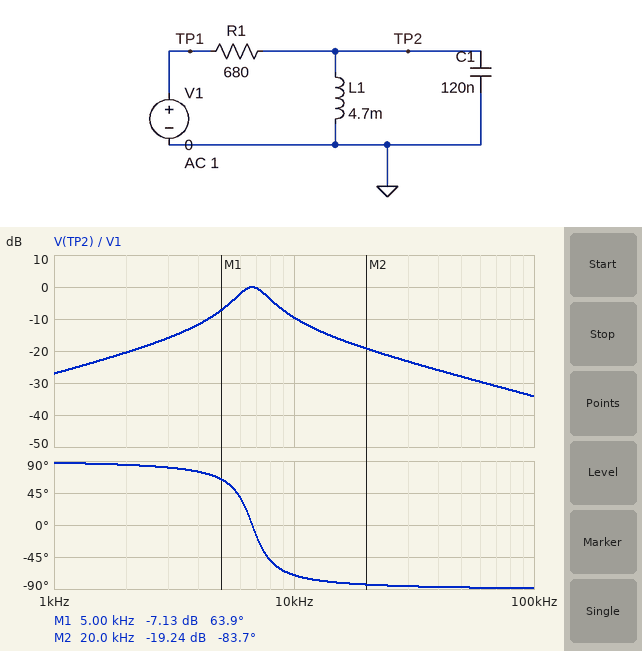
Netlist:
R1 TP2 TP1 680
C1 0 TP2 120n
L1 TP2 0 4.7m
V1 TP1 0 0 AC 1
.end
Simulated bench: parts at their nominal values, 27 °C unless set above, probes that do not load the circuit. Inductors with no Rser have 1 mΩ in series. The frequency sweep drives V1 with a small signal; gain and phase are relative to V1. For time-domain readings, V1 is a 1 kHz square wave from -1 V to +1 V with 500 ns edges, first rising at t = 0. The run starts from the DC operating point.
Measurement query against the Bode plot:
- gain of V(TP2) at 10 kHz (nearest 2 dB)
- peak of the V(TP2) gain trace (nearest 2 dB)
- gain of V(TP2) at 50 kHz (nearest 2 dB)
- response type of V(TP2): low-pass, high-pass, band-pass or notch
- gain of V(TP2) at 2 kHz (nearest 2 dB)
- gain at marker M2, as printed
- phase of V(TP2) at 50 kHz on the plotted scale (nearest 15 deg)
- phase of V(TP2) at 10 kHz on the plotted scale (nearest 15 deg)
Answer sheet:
-10 dB
0 dB
-28 dB
band-pass
-20 dB
-19.24 dB
-90 deg
-75 deg
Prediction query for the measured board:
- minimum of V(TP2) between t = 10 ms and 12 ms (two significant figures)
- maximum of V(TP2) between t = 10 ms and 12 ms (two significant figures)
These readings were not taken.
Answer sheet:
-480 mV
480 mV
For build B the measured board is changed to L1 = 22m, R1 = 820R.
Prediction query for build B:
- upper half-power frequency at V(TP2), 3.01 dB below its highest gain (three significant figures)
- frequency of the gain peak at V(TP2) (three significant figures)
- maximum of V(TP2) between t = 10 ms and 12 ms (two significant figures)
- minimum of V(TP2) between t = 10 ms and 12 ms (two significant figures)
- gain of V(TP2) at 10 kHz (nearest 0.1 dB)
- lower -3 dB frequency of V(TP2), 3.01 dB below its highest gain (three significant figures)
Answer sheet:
4.01 kHz
3.10 kHz
800 mV
-800 mV
-15.1 dB
2.39 kHz
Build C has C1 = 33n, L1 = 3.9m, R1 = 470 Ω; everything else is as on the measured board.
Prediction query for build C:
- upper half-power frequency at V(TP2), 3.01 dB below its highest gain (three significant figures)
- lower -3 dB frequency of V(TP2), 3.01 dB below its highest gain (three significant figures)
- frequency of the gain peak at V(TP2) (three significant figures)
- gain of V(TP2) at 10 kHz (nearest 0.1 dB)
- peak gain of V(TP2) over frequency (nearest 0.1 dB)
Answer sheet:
20.1 kHz
9.81 kHz
14.0 kHz
-2.8 dB
0 dB
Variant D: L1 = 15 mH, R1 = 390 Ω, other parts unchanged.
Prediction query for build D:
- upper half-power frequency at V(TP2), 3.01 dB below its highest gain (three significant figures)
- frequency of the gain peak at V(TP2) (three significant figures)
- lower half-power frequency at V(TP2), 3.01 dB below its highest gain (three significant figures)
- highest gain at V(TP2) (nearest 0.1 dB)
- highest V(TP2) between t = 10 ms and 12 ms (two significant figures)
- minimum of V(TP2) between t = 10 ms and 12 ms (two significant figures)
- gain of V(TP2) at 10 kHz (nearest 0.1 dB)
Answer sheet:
5.82 kHz
3.75 kHz
2.42 kHz
0 dB
1.0 V
-1.0 V
-8.7 dB
